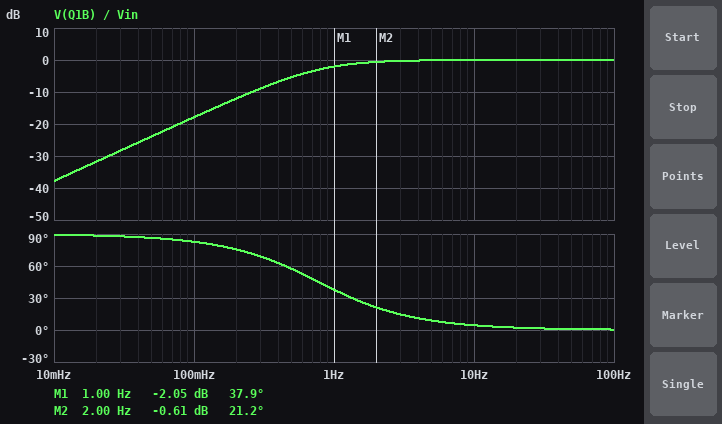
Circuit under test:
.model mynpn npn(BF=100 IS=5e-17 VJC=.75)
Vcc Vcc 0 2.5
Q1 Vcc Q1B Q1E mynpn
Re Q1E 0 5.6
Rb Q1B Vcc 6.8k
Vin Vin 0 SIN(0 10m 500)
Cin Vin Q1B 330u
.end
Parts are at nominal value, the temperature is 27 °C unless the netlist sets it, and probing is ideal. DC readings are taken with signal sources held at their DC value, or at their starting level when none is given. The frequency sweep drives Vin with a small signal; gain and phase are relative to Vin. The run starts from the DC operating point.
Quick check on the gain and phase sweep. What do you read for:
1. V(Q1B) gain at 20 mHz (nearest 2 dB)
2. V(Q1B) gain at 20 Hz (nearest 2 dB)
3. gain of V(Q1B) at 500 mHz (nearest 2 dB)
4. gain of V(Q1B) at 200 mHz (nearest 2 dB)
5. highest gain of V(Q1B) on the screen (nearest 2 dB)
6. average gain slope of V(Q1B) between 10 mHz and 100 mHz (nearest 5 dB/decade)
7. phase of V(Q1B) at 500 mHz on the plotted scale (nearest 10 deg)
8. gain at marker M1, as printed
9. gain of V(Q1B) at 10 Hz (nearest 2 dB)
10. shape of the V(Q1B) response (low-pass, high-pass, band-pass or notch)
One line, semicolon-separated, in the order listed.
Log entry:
-32 dB; 0 dB; -6 dB; -12 dB; 0 dB; 20 dB/decade; 60 deg; -2.05 dB; 0 dB; high-pass
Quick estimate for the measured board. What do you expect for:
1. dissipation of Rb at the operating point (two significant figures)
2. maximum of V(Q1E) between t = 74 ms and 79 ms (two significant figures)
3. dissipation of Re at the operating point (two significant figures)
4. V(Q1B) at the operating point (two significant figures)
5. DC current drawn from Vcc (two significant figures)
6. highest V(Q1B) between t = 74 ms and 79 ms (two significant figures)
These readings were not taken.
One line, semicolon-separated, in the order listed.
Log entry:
330 µW; 130 mV; 2.8 mW; 1.0 V; 22 mA; 1.0 V
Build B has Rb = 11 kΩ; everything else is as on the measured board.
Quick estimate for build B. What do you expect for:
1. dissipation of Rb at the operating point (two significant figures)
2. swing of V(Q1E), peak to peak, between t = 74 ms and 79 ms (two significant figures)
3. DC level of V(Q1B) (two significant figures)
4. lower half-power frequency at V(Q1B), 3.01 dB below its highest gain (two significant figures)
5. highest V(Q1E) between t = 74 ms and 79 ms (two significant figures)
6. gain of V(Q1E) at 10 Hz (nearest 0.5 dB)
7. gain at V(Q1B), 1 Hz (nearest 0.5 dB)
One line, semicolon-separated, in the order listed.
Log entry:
220 µW; 15 mV; 940 mV; 690 mHz; 88 mV; -2.5 dB; -1.5 dB
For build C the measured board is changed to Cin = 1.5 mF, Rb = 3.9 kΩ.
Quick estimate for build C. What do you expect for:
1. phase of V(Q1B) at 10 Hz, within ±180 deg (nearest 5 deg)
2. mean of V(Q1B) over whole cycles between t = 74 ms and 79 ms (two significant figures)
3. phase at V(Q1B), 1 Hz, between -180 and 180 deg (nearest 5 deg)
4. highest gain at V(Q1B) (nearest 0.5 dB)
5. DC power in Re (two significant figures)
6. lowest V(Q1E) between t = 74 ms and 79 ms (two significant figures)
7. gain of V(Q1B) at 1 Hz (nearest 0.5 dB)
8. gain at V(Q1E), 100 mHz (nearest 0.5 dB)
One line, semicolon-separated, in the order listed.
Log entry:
0 deg; 1.1 V; 10 deg; 0 dB; 7.5 mW; 200 mV; 0 dB; -8.0 dB
